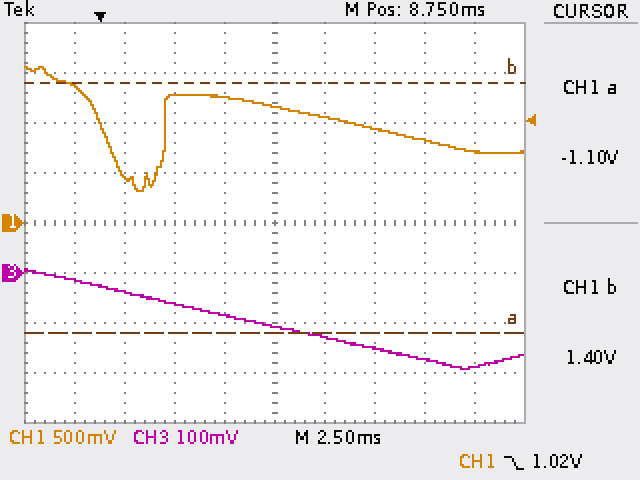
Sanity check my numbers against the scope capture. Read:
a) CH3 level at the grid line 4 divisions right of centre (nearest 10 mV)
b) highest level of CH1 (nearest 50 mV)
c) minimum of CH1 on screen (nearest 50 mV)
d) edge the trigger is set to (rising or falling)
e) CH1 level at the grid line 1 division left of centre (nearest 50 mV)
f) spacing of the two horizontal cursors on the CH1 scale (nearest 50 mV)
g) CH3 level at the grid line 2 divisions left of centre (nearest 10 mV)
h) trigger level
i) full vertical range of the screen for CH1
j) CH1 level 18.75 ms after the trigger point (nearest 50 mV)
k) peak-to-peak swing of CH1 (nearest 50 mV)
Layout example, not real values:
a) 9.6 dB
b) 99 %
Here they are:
a) -190 mV
b) 1.55 V
c) 300 mV
d) falling
e) 1.25 V
f) 2.50 V
g) -60 mV
h) 1.02 V
i) 4 V
j) 700 mV
k) 1.25 V
